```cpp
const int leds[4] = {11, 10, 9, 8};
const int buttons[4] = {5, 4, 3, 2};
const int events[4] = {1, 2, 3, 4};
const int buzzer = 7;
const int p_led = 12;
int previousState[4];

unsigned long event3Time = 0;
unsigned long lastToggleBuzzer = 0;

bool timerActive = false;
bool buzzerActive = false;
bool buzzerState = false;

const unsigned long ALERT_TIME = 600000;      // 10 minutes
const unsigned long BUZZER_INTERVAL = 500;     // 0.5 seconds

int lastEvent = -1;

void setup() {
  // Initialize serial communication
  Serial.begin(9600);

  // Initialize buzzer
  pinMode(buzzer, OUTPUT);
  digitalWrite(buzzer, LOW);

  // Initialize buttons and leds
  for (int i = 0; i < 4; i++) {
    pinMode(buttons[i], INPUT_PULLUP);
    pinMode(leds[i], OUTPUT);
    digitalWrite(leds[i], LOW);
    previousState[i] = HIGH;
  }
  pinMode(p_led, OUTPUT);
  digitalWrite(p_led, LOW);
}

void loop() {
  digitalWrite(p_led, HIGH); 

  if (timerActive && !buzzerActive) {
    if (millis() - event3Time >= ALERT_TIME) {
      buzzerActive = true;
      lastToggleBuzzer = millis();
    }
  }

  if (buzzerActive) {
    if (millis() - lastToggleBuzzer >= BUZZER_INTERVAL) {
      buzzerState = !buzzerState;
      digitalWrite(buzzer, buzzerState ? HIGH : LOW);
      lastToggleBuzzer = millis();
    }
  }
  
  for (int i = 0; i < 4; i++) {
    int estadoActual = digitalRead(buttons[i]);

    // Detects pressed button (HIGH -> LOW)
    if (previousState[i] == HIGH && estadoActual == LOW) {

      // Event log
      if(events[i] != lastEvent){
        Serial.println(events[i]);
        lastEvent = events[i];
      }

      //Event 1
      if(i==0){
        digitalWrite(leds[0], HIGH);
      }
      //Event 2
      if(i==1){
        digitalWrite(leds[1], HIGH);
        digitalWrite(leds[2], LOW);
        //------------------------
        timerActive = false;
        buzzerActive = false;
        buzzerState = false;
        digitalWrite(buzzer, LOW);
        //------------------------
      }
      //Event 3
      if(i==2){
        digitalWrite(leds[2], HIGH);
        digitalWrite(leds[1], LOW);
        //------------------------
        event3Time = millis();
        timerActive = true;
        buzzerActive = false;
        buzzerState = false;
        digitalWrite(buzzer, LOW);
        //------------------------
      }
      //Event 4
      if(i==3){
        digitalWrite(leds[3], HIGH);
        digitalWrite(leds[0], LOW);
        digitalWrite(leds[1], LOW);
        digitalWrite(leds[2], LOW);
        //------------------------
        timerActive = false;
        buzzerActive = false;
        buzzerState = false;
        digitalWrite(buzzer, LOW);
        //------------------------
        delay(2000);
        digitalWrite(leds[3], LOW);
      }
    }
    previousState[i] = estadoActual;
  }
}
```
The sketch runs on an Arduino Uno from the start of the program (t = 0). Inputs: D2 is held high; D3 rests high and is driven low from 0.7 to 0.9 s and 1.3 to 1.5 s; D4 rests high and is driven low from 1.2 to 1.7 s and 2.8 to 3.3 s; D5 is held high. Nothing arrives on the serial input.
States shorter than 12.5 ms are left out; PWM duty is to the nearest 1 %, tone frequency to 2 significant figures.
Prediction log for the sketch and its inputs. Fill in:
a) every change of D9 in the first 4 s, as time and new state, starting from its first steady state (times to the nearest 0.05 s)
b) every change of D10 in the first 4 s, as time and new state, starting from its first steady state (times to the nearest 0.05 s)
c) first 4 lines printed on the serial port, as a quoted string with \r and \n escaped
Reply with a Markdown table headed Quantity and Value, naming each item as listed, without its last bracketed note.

| Quantity | Value |
|---|---|
| every change of D9 in the first 4 s, as time and new state, starting from its first steady state | 0 s low; 0.7 s high; 1.2 s low; 1.3 s high; 2.8 s low |
| every change of D10 in the first 4 s, as time and new state, starting from its first steady state | 0 s low; 1.2 s high; 1.3 s low; 2.8 s high |
| first 4 lines printed on the serial port, as a quoted string with \r and \n escaped | "3\r\n2\r\n3\r\n2\r\n" |
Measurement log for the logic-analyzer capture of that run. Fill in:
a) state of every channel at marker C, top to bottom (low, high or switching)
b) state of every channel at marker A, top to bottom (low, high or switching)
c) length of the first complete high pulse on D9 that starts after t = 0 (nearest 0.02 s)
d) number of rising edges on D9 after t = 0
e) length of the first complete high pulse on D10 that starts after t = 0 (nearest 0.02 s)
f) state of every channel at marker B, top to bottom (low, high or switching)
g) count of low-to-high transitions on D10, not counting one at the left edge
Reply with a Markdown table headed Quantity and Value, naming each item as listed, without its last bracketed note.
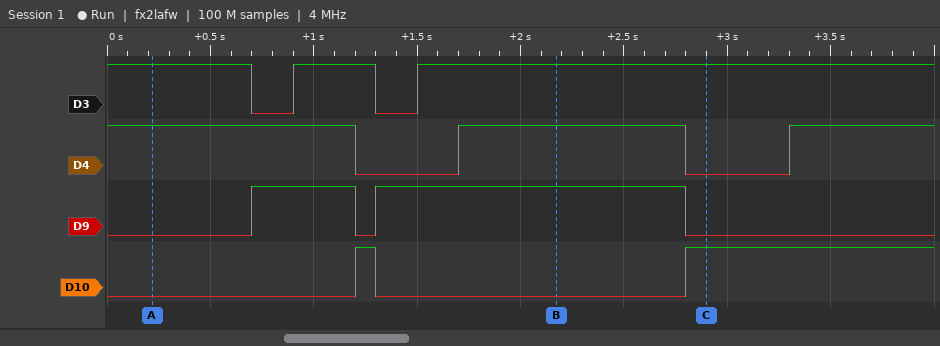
| Quantity | Value |
|---|---|
| state of every channel at marker C, top to bottom | D3 high, D4 low, D9 low, D10 high |
| state of every channel at marker A, top to bottom | D3 high, D4 high, D9 low, D10 low |
| length of the first complete high pulse on D9 that starts after t = 0 | 0.50 s |
| number of rising edges on D9 after t = 0 | 2 |
| length of the first complete high pulse on D10 that starts after t = 0 | 0.10 s |
| state of every channel at marker B, top to bottom | D3 high, D4 high, D9 high, D10 low |
| count of low-to-high transitions on D10, not counting one at the left edge | 2 |
